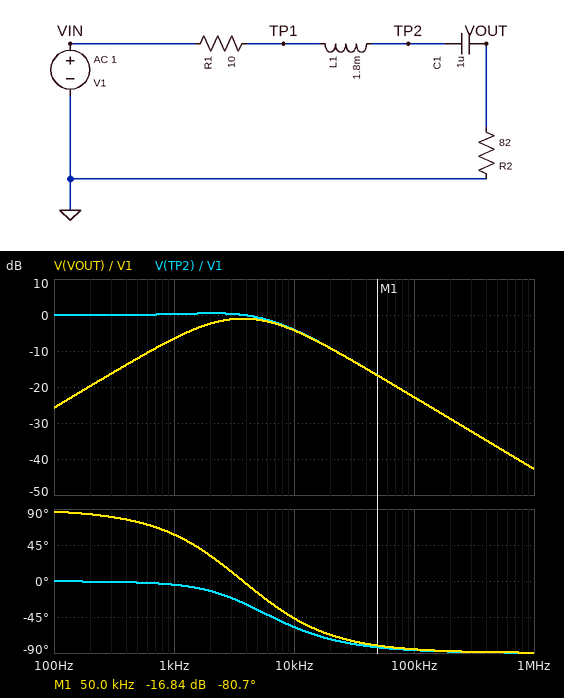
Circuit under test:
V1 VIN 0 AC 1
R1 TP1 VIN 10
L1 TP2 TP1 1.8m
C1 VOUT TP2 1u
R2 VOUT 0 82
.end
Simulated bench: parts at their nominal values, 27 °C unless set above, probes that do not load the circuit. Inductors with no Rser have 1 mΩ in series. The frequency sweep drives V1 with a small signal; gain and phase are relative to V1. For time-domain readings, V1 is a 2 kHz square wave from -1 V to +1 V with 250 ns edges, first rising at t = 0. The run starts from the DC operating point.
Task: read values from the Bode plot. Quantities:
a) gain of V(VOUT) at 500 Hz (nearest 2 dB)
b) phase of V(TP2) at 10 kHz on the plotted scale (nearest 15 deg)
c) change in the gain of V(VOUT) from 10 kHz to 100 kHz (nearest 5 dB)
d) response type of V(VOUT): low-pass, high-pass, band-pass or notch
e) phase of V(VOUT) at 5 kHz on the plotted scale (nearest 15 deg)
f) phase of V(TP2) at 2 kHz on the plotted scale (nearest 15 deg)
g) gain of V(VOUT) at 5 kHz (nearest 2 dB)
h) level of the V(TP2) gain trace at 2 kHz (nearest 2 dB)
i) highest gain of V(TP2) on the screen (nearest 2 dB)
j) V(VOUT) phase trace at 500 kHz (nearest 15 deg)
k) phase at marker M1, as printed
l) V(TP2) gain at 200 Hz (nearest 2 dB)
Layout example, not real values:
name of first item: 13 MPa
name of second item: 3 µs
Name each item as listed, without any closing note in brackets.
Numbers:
gain of V(VOUT) at 500 Hz: -12 dB
phase of V(TP2) at 10 kHz on the plotted scale: -60 deg
change in the gain of V(VOUT) from 10 kHz to 100 kHz: -20 dB
response type of V(VOUT): low-pass, high-pass, band-pass or notch: band-pass
phase of V(VOUT) at 5 kHz on the plotted scale: -15 deg
phase of V(TP2) at 2 kHz on the plotted scale: -15 deg
gain of V(VOUT) at 5 kHz: -2 dB
level of the V(TP2) gain trace at 2 kHz: 0 dB
highest gain of V(TP2) on the screen: 0 dB
V(VOUT) phase trace at 500 kHz: -90 deg
phase at marker M1, as printed: -80.7 deg
V(TP2) gain at 200 Hz: 0 dB
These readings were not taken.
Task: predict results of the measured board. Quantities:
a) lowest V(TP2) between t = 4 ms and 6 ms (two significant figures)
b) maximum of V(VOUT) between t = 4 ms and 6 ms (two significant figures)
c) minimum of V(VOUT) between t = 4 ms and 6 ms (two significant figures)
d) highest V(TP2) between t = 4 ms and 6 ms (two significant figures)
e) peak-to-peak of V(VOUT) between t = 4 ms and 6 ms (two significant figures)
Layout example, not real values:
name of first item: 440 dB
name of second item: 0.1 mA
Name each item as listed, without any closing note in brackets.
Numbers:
lowest V(TP2) between t = 4 ms and 6 ms: -1.1 V
maximum of V(VOUT) between t = 4 ms and 6 ms: 1.3 V
minimum of V(VOUT) between t = 4 ms and 6 ms: -1.3 V
highest V(TP2) between t = 4 ms and 6 ms: 1.1 V
peak-to-peak of V(VOUT) between t = 4 ms and 6 ms: 2.6 V
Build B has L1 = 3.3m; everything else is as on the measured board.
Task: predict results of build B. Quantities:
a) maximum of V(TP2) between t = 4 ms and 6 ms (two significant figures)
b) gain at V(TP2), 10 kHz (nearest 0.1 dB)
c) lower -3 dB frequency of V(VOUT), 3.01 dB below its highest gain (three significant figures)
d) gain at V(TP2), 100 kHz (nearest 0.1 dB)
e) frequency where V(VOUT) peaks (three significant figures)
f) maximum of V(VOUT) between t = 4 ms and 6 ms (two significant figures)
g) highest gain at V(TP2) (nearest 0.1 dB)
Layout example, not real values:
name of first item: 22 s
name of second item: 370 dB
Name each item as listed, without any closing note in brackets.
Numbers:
maximum of V(TP2) between t = 4 ms and 6 ms: 1.3 V
gain at V(TP2), 10 kHz: -8.1 dB
lower -3 dB frequency of V(VOUT), 3.01 dB below its highest gain: 1.33 kHz
gain at V(TP2), 100 kHz: -28.1 dB
frequency where V(VOUT) peaks: 2.77 kHz
maximum of V(VOUT) between t = 4 ms and 6 ms: 1.2 V
highest gain at V(TP2): 1.2 dB
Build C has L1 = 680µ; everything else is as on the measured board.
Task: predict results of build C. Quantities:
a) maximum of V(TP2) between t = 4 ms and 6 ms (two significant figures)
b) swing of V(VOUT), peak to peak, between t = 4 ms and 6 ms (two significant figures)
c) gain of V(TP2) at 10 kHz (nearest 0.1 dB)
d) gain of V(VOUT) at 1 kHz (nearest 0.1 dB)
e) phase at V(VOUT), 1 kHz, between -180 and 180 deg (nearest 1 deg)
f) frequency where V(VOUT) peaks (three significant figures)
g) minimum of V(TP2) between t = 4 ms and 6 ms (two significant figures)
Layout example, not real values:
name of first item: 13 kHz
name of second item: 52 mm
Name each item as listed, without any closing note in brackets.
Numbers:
maximum of V(TP2) between t = 4 ms and 6 ms: 1.0 V
swing of V(VOUT), peak to peak, between t = 4 ms and 6 ms: 2.9 V
gain of V(TP2) at 10 kHz: -1.2 dB
gain of V(VOUT) at 1 kHz: -6.8 dB
phase at V(VOUT), 1 kHz, between -180 and 180 deg: 59 deg
frequency where V(VOUT) peaks: 6.10 kHz
minimum of V(TP2) between t = 4 ms and 6 ms: -1.0 V
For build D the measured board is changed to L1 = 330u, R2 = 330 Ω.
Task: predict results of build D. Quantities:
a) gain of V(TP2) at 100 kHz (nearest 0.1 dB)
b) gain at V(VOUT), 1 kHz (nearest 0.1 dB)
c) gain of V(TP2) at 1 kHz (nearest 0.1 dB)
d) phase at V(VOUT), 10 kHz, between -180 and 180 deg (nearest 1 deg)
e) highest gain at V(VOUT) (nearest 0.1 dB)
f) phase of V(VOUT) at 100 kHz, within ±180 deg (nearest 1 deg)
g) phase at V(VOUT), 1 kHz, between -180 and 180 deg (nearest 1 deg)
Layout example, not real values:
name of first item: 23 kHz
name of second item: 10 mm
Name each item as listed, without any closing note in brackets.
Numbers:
gain of V(TP2) at 100 kHz: -1.6 dB
gain at V(VOUT), 1 kHz: -1.1 dB
gain of V(TP2) at 1 kHz: -0.2 dB
phase at V(VOUT), 10 kHz, between -180 and 180 deg: -1 deg
highest gain at V(VOUT): -0.3 dB
phase of V(VOUT) at 100 kHz, within ±180 deg: -31 deg
phase at V(VOUT), 1 kHz, between -180 and 180 deg: 25 deg
